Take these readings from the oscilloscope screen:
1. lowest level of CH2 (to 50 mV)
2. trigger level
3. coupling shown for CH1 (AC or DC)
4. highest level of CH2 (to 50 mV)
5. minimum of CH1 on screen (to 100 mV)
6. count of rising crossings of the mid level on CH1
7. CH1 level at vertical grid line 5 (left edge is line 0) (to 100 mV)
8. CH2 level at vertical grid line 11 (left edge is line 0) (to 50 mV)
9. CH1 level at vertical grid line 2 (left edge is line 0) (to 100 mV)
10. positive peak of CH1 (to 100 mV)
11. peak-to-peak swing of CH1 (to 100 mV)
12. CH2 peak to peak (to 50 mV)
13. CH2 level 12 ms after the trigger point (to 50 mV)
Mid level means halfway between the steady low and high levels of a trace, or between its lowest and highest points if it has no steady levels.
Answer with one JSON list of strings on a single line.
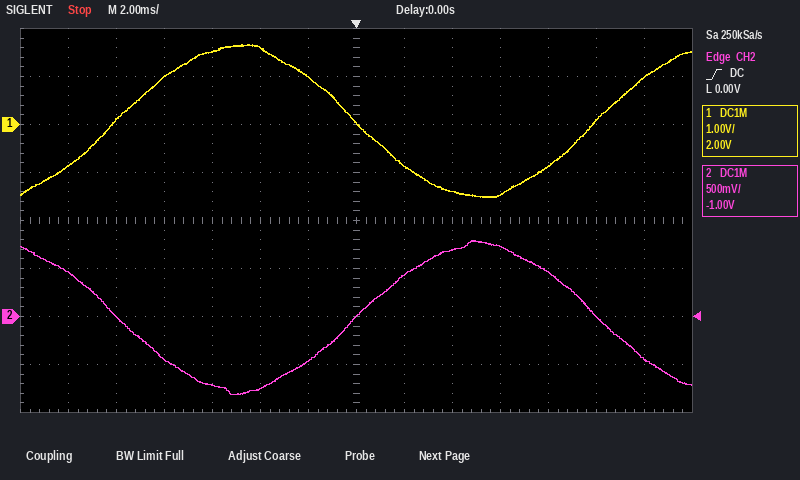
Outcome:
["-800 mV", "0.00 V", "DC", "800 mV", "-1.5 V", "2", "1.6 V", "450 mV", "100 mV", "1.7 V", "3.2 V", "1.60 V", "-450 mV"]
